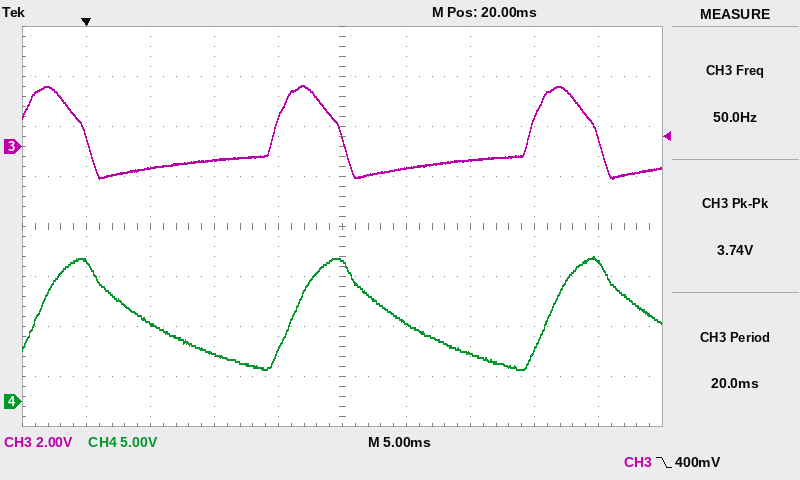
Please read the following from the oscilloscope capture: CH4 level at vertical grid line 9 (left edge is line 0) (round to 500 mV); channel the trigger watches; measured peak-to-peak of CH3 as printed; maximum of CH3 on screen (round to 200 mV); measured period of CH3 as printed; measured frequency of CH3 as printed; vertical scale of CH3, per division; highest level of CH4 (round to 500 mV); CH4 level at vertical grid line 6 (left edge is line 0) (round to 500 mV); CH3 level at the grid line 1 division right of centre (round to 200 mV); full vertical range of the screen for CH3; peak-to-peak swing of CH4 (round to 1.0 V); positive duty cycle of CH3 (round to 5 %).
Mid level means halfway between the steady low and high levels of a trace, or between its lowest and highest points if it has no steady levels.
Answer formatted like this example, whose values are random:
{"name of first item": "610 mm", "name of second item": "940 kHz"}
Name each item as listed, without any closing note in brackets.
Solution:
{"CH4 level at vertical grid line 9 (left edge is line 0)": "14.0 V", "channel the trigger watches": "CH3", "measured peak-to-peak of CH3 as printed": "3.74 V", "maximum of CH3 on screen": "2.4 V", "measured period of CH3 as printed": "20.0 ms", "measured frequency of CH3 as printed": "50.0 Hz", "vertical scale of CH3, per division": "2 V", "highest level of CH4": "14.5 V", "CH4 level at vertical grid line 6 (left edge is line 0)": "8.0 V", "CH3 level at the grid line 1 division right of centre": "-800 mV", "full vertical range of the screen for CH3": "16 V", "peak-to-peak swing of CH4": "11.0 V", "positive duty cycle of CH3": "25 %"}
